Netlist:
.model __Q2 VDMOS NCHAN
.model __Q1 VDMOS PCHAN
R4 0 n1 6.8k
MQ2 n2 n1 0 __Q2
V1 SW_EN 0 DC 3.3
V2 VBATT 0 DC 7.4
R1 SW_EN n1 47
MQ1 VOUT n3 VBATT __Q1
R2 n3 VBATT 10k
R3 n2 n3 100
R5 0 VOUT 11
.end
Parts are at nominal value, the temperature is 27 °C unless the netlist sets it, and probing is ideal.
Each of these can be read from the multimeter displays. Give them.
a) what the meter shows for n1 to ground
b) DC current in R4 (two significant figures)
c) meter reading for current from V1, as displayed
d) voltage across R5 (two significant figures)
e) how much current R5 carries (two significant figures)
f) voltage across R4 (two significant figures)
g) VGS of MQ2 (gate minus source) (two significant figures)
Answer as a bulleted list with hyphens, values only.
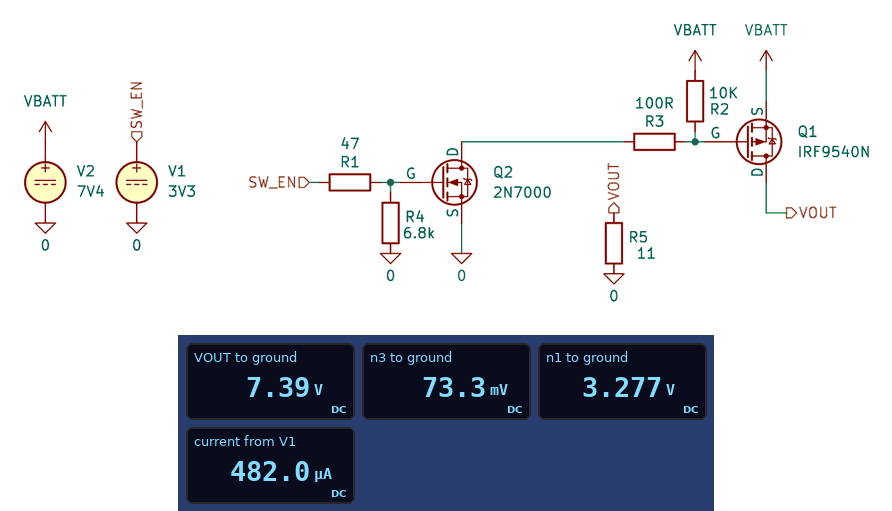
- 3.277 V
- 480 µA
- 482.0 µA
- 7.4 V
- 670 mA
- 3.3 V
- 3.3 V
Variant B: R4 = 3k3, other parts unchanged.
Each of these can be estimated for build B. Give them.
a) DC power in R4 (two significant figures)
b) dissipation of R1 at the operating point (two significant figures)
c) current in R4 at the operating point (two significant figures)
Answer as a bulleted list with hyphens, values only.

- 3.2 mW
- 46 µW
- 990 µA
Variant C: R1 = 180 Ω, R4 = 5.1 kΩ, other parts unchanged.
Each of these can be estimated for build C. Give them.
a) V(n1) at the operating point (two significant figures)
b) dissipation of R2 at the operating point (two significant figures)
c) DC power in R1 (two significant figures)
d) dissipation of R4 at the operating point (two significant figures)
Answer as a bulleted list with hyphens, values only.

- 3.2 V
- 5.4 mW
- 70 µW
- 2.0 mW
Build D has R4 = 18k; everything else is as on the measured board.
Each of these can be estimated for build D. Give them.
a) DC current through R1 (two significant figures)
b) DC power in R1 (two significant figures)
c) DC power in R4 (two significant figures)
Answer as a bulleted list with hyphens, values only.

- 180 µA
- 1.6 µW
- 600 µW
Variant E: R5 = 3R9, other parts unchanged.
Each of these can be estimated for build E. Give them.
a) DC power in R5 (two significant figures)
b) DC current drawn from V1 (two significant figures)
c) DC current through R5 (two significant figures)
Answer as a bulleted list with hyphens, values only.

- 14 W
- 480 µA
- 1.9 A
